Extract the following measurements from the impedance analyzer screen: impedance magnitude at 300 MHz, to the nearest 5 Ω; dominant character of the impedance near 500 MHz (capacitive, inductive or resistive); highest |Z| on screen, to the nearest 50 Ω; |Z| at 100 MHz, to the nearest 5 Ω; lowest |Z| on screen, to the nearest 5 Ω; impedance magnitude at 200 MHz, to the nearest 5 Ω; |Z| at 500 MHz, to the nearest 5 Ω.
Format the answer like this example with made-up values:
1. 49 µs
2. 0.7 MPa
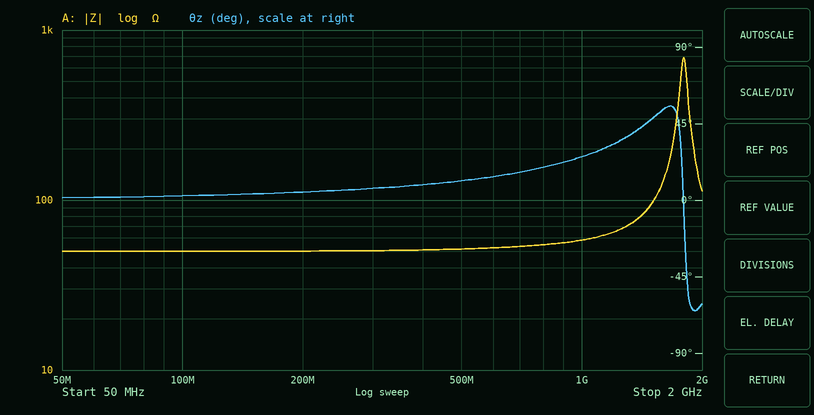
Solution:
1. 50 Ω
2. resistive
3. 700 Ω
4. 50 Ω
5. 50 Ω
6. 50 Ω
7. 50 Ω
